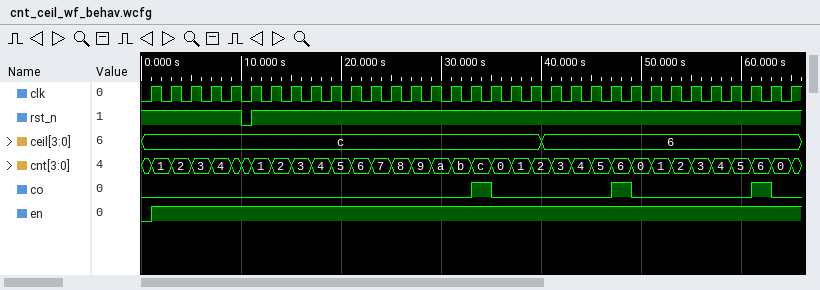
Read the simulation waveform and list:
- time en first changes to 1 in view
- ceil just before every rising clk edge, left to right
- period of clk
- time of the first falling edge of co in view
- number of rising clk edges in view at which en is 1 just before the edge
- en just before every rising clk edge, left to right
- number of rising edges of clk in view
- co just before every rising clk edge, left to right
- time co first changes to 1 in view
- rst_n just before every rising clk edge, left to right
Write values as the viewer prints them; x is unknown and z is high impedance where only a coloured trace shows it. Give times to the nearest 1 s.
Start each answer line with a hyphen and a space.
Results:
- 1 s
- c, c, c, c, c, c, c, c, c, c, c, c, c, c, c, c, c, c, c, c, 6, 6, 6, 6, 6, 6, 6, 6, 6, 6, 6, 6, 6
- 2 s
- 35 s
- 32
- 0 1 1 1 1 1 1 1 1 1 1 1 1 1 1 1 1 1 1 1 1 1 1 1 1 1 1 1 1 1 1 1 1
- 33
- 0 0 0 0 0 0 0 0 0 0 0 0 0 0 0 0 0 1 0 0 0 0 0 0 1 0 0 0 0 0 0 1 0
- 33 s
- 1 1 1 1 1 0 1 1 1 1 1 1 1 1 1 1 1 1 1 1 1 1 1 1 1 1 1 1 1 1 1 1 1
